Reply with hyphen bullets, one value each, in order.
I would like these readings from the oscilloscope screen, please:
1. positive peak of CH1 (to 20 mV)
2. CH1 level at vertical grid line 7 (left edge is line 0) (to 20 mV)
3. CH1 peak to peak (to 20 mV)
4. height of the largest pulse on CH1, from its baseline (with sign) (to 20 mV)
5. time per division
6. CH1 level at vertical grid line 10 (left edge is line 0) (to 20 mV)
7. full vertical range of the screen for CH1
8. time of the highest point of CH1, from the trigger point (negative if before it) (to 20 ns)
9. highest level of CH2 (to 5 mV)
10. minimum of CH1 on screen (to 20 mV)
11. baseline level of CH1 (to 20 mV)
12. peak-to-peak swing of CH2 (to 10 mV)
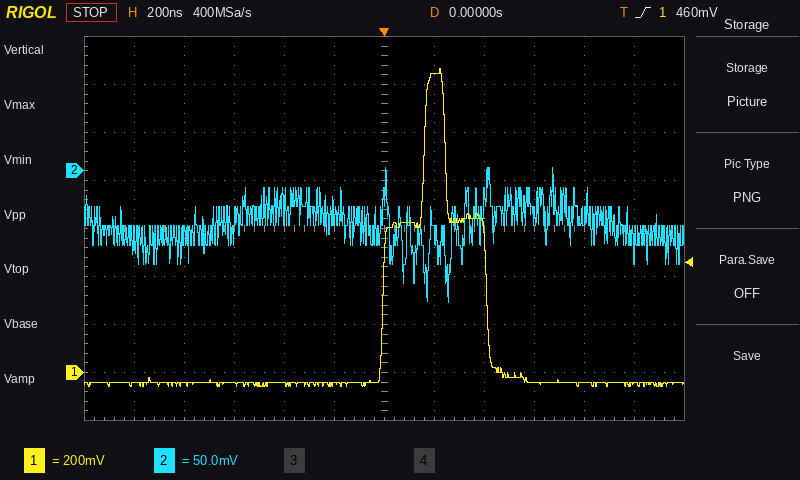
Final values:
- 1.26 V
- 1.24 V
- 1.32 V
- +1.30 V
- 200 ns
- -40 mV
- 1.6 V
- +220 ns
- 5 mV
- -60 mV
- -40 mV
- 140 mV
